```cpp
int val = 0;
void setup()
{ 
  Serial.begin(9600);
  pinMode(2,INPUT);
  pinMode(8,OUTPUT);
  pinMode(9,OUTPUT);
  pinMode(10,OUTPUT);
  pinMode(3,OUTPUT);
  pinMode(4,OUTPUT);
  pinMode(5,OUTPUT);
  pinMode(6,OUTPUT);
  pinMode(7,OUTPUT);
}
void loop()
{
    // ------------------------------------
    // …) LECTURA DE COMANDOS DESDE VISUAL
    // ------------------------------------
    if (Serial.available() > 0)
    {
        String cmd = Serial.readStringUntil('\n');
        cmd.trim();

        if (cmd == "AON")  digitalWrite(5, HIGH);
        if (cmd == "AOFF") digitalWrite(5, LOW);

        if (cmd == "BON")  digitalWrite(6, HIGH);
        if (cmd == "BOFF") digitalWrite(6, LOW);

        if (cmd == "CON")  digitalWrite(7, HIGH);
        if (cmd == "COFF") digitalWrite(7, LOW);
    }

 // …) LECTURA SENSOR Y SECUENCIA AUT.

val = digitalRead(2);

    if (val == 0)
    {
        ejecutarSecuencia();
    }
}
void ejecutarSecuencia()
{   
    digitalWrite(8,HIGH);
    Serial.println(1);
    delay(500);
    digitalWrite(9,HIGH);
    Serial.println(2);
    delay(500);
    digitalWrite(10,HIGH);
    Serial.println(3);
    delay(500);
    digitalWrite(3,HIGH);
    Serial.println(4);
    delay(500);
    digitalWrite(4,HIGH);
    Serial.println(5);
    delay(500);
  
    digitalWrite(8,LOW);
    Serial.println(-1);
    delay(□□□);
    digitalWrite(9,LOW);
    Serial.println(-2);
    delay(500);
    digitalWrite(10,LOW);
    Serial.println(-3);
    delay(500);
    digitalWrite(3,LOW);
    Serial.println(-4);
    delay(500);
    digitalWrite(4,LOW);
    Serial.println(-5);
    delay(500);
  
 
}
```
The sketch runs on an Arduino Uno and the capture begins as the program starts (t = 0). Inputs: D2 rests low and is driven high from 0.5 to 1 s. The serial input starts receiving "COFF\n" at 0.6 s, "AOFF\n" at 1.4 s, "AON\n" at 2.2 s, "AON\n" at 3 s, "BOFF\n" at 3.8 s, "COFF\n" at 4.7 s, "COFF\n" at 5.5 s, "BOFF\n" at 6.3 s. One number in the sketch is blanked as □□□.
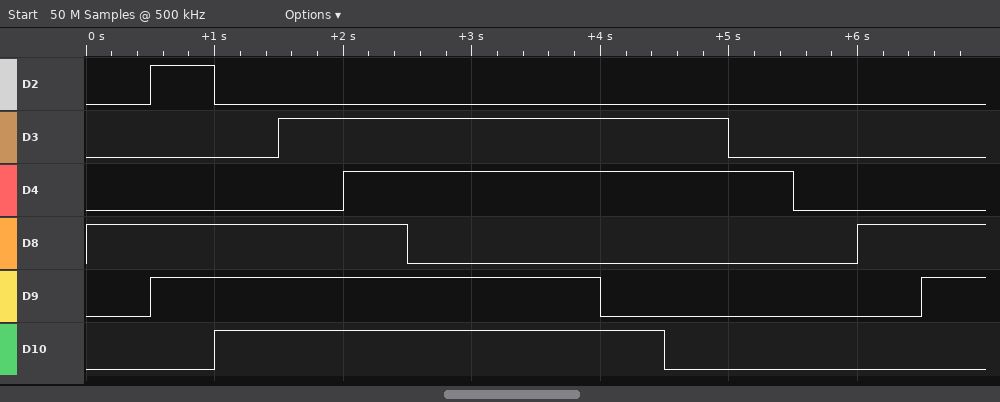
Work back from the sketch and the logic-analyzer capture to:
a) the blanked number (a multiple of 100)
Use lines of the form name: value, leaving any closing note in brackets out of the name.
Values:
the blanked number: 1500
